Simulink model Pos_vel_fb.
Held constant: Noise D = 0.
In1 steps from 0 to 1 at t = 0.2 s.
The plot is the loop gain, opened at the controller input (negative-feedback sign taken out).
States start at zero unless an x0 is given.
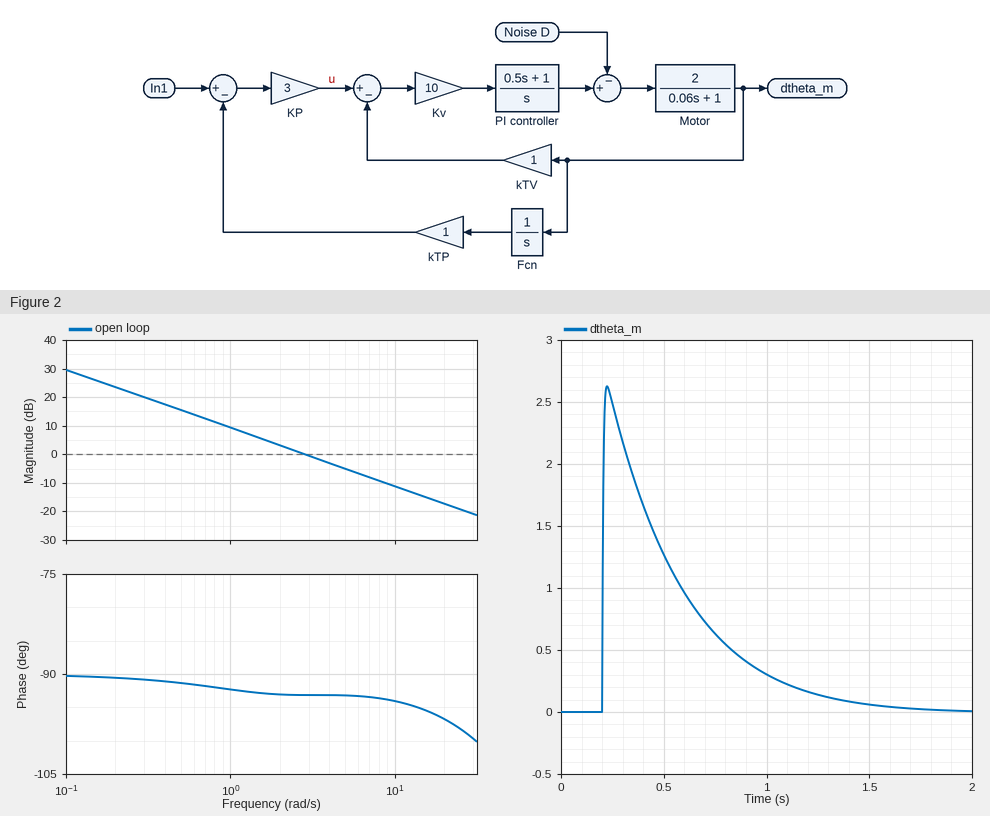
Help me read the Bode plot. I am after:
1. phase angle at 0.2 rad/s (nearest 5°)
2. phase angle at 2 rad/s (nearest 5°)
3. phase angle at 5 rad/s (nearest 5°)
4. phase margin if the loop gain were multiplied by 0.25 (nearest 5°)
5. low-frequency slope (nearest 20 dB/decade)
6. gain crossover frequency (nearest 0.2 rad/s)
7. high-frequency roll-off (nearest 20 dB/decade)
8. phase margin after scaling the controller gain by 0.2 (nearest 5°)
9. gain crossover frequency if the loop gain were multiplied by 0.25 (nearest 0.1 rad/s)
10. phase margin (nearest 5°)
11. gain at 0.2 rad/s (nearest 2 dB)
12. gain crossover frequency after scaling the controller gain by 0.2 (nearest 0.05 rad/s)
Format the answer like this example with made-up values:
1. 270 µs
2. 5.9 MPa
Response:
1. -90°
2. -95°
3. -95°
4. 90°
5. -20 dB/decade
6. 2.8 rad/s
7. -20 dB/decade
8. 90°
9. 0.7 rad/s
10. 85°
11. 24 dB
12. 0.60 rad/s
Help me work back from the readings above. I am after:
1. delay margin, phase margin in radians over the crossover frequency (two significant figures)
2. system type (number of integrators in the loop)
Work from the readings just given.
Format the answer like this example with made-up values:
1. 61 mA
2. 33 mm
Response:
1. 0.53 s
2. 1
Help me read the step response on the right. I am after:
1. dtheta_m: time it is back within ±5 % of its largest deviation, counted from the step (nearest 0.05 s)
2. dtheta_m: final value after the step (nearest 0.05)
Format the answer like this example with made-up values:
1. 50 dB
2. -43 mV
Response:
1. 1.05 s
2. 0.00
